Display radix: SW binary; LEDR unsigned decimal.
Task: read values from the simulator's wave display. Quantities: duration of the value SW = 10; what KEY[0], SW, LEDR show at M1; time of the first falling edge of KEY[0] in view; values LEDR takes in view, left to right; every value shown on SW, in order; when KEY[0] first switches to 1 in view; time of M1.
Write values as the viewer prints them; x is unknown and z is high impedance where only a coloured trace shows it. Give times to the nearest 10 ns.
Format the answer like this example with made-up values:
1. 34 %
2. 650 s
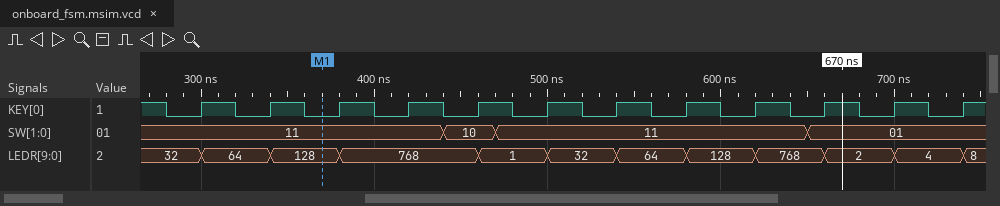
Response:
1. 30 ns
2. KEY[0]=0, SW=11, LEDR=128
3. 280 ns
4. 32, 64, 128, 768, 1, 32, 64, 128, 768, 2, 4, 8
5. 11, 10, 11, 01
6. 300 ns
7. 370 ns
